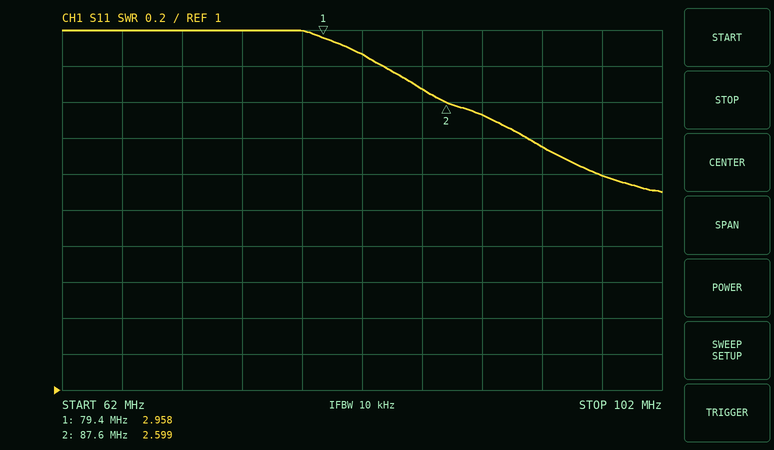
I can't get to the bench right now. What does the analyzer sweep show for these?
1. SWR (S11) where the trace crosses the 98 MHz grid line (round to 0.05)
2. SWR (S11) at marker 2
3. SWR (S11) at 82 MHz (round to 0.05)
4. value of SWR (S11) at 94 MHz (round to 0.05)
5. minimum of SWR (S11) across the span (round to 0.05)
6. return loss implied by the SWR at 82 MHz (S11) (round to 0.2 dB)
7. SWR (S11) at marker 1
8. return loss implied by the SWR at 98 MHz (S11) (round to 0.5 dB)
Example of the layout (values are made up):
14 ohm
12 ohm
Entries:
2.20
2.599
2.85
2.35
2.10
6.4 dB
2.958
8.5 dB
